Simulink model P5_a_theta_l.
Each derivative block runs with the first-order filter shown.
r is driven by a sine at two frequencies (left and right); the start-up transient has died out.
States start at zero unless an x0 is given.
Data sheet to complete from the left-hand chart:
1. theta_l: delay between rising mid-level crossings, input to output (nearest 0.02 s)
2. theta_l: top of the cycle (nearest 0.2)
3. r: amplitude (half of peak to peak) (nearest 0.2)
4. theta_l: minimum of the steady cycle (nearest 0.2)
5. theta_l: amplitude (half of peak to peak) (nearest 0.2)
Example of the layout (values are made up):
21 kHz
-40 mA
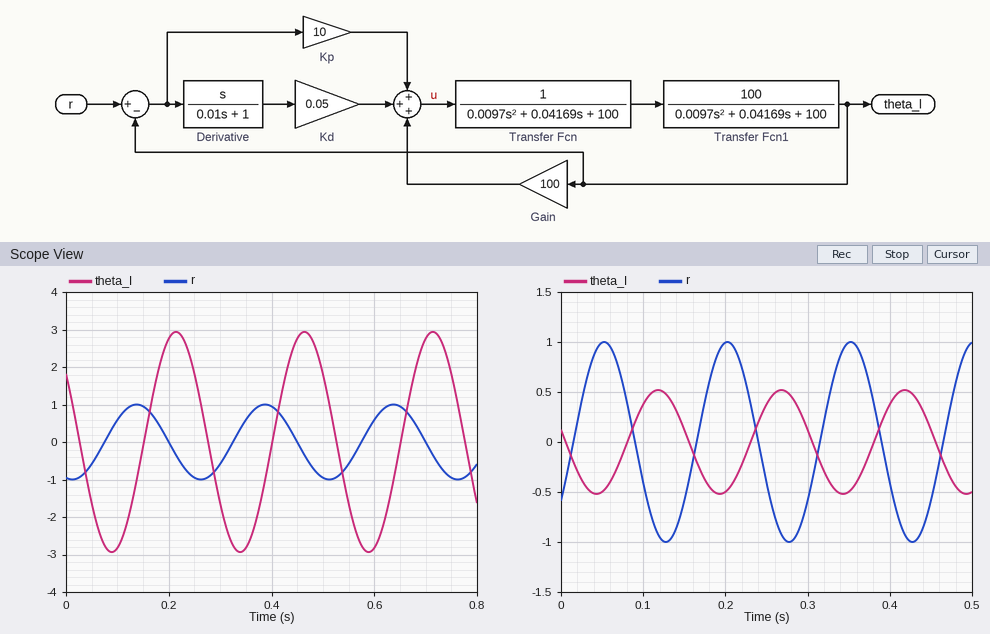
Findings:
0.08 s
3.0
1.0
-3.0
3.0
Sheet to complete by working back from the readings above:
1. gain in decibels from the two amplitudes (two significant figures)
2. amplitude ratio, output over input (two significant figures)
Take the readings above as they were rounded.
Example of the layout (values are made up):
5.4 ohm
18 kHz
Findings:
9.5 dB
3.0
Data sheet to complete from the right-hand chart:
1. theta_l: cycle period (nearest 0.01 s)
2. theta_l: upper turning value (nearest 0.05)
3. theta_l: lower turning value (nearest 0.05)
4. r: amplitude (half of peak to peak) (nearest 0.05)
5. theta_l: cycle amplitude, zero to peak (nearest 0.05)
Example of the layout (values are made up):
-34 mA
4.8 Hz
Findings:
0.15 s
0.50
-0.50
1.00
0.50
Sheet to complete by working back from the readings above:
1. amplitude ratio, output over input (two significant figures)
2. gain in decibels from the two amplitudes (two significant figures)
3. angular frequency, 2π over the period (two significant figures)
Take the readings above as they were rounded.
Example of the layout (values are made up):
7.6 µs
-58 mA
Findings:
0.50
-6.0 dB
42 rad/s
